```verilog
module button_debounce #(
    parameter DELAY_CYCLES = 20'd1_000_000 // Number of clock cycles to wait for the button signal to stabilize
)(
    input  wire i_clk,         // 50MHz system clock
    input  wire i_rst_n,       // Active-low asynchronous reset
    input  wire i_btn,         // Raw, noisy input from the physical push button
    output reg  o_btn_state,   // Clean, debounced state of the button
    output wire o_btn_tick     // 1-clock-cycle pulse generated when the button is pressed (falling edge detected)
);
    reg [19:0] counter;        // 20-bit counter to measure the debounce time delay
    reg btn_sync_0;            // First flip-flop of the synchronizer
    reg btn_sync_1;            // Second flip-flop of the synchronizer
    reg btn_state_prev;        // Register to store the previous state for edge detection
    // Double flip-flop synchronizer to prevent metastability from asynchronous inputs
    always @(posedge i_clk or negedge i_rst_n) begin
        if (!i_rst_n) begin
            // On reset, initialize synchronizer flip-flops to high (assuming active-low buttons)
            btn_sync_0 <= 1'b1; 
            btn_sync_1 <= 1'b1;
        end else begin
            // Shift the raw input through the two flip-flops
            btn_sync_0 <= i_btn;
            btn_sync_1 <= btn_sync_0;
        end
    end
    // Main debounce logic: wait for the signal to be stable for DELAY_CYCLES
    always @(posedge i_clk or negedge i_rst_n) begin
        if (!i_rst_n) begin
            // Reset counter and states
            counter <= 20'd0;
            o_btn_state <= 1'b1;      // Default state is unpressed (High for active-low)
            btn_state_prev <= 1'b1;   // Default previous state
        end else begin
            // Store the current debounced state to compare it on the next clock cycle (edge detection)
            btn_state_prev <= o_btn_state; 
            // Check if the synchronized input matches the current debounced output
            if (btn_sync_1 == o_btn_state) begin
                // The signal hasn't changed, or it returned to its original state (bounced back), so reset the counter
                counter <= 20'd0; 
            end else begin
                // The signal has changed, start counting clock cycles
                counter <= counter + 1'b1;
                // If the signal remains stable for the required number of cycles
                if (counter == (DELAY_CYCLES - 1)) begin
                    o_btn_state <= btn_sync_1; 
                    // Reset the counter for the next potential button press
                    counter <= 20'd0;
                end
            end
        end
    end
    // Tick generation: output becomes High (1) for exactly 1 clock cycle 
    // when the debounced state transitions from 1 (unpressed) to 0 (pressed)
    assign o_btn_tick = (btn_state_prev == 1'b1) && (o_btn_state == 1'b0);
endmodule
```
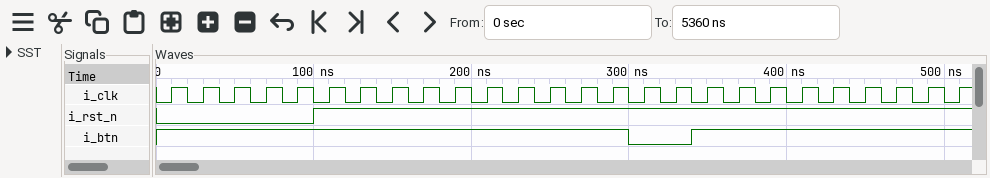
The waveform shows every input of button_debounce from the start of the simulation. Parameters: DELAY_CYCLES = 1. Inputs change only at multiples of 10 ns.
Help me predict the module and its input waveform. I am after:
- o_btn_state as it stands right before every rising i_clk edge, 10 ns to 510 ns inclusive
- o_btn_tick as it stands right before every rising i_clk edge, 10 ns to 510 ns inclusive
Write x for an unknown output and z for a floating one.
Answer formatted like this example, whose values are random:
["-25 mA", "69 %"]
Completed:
["1 1 1 1 1 1 1 1 1 1 1 1 1 1 1 1 1 1 0 0 1 1 1 1 1 1", "0 0 0 0 0 0 0 0 0 0 0 0 0 0 0 0 0 0 1 0 0 0 0 0 0 0"]
